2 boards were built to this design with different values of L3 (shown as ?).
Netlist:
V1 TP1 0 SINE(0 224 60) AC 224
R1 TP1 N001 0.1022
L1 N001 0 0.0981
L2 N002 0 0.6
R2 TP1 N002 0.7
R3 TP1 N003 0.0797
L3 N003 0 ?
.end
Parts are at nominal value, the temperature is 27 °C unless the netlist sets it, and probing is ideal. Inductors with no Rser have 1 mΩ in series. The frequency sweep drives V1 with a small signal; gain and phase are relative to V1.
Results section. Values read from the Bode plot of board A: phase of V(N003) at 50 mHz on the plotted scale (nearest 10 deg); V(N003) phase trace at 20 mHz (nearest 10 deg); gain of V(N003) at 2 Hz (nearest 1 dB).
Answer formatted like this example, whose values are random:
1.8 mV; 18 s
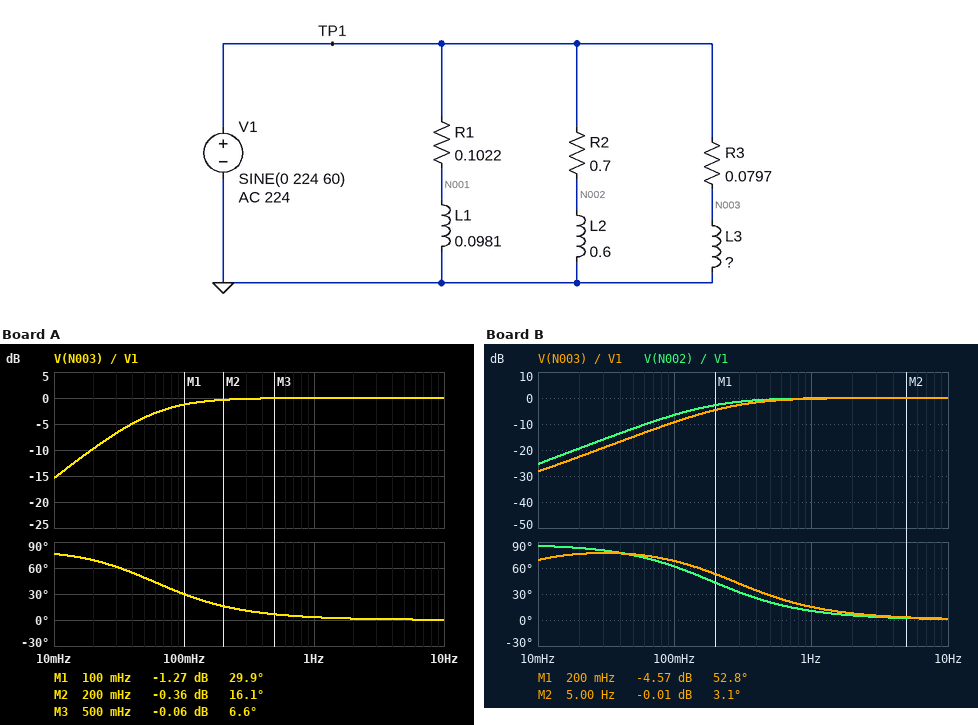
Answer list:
50 deg; 70 deg; 0 dB
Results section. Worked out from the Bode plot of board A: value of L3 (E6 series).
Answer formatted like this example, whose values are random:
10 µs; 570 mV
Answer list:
220 mH
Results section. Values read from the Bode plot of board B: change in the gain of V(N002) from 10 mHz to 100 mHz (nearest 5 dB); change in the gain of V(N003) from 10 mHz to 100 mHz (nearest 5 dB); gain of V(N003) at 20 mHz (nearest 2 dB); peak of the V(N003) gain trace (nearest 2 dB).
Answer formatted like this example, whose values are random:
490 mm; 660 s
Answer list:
20 dB; 20 dB; -22 dB; 0 dB
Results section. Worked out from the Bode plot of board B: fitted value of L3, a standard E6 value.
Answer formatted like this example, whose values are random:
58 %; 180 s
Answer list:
47 mH
